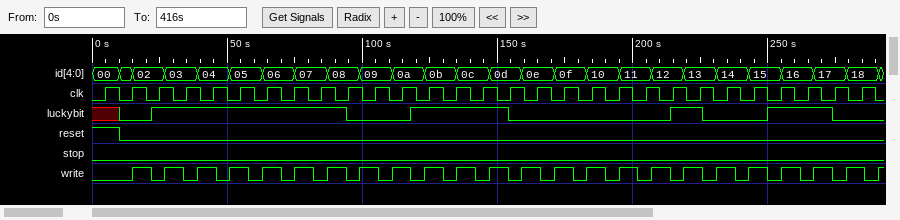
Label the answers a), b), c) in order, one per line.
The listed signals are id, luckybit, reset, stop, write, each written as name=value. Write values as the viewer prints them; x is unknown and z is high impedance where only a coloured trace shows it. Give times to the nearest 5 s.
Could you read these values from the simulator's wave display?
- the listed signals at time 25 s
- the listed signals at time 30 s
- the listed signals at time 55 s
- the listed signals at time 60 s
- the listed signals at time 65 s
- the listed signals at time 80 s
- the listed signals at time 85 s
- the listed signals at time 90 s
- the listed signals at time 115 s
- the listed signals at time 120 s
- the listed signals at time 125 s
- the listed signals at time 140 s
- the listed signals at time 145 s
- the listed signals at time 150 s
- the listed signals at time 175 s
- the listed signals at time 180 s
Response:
a) id=02, luckybit=1, reset=0, stop=0, write=0
b) id=03, luckybit=1, reset=0, stop=0, write=1
c) id=05, luckybit=1, reset=0, stop=0, write=1
d) id=05, luckybit=1, reset=0, stop=0, write=0
e) id=06, luckybit=1, reset=0, stop=0, write=1
f) id=07, luckybit=1, reset=0, stop=0, write=1
g) id=07, luckybit=1, reset=0, stop=0, write=0
h) id=08, luckybit=1, reset=0, stop=0, write=1
i) id=0a, luckybit=0, reset=0, stop=0, write=1
j) id=0a, luckybit=1, reset=0, stop=0, write=0
k) id=0b, luckybit=1, reset=0, stop=0, write=1
l) id=0c, luckybit=1, reset=0, stop=0, write=1
m) id=0c, luckybit=1, reset=0, stop=0, write=0
n) id=0d, luckybit=1, reset=0, stop=0, write=1
o) id=0f, luckybit=0, reset=0, stop=0, write=1
p) id=0f, luckybit=0, reset=0, stop=0, write=0
